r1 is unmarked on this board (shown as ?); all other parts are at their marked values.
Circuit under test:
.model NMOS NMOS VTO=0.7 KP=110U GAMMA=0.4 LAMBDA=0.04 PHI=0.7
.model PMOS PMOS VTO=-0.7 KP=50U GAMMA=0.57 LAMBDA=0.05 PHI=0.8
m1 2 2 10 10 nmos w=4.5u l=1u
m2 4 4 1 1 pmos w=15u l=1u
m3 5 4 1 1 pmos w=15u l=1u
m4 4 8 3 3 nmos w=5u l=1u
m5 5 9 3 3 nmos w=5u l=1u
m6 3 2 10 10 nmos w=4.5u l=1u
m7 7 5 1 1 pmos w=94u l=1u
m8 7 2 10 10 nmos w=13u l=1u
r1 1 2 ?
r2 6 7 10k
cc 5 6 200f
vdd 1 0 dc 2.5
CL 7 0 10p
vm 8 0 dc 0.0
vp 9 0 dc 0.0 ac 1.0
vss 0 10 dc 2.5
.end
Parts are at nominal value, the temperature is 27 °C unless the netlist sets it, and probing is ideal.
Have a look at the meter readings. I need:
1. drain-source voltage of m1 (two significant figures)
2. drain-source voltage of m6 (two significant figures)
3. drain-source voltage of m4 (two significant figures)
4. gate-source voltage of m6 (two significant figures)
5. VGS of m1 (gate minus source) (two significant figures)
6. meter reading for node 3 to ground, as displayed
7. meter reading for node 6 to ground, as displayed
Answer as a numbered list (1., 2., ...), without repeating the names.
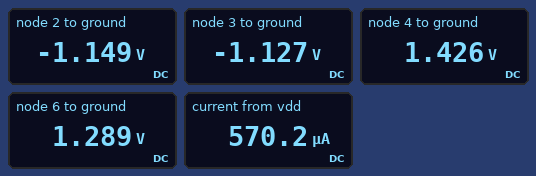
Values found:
1. 1.4 V
2. 1.4 V
3. 2.6 V
4. 1.4 V
5. 1.4 V
6. -1.127 V
7. 1.289 V
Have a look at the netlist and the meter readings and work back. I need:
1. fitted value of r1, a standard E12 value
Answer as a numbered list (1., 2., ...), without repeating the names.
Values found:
1. 33 kΩ
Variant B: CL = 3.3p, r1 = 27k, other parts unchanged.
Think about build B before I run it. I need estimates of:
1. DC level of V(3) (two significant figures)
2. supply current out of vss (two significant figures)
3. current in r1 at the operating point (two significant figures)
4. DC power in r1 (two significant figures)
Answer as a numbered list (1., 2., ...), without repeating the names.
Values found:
1. -1.2 V
2. 680 µA
3. 130 µA
4. 480 µW
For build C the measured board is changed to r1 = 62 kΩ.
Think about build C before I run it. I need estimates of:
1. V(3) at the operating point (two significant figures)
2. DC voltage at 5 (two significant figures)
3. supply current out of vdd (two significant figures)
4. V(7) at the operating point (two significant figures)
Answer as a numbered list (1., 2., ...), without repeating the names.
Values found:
1. -1.0 V
2. 1.5 V
3. 320 µA
4. 1.4 V
